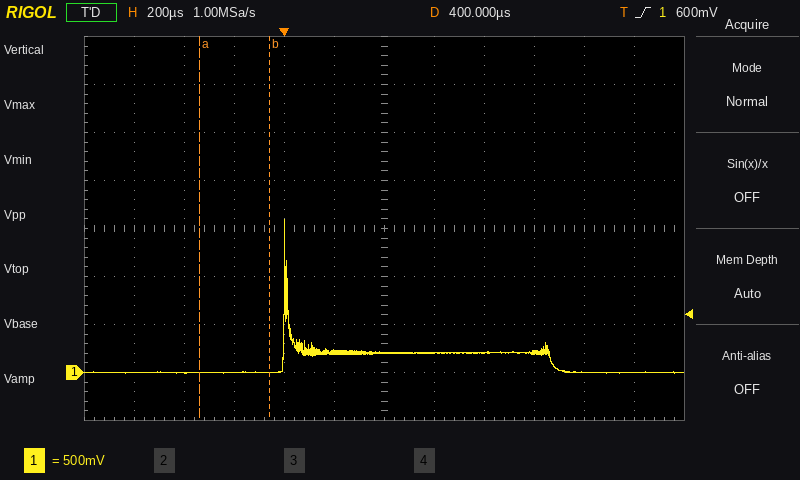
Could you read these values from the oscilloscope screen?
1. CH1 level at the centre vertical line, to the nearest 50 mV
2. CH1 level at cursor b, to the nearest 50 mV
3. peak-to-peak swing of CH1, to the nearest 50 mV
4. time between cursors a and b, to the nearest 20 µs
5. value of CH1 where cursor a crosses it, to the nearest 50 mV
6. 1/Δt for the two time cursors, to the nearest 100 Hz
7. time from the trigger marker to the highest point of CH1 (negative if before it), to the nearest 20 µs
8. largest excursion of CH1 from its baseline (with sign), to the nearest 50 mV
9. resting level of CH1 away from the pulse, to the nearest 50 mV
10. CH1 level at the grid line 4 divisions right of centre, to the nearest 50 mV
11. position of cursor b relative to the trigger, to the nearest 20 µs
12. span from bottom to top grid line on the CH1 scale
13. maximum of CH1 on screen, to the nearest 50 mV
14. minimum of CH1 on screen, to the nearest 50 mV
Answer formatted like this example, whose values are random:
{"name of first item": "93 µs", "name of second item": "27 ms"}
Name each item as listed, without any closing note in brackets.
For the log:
{"CH1 level at the centre vertical line, to the nearest 50 mV": "200 mV", "CH1 level at cursor b, to the nearest 50 mV": "0 mV", "peak-to-peak swing of CH1, to the nearest 50 mV": "1.60 V", "time between cursors a and b, to the nearest 20 µs": "280 µs", "value of CH1 where cursor a crosses it, to the nearest 50 mV": "0 mV", "1/Δt for the two time cursors, to the nearest 100 Hz": "3.6 kHz", "time from the trigger marker to the highest point of CH1 (negative if before it), to the nearest 20 µs": "0 µs", "largest excursion of CH1 from its baseline (with sign), to the nearest 50 mV": "+1.60 V", "resting level of CH1 away from the pulse, to the nearest 50 mV": "0 mV", "CH1 level at the grid line 4 divisions right of centre, to the nearest 50 mV": "0 mV", "position of cursor b relative to the trigger, to the nearest 20 µs": "-60 µs", "span from bottom to top grid line on the CH1 scale": "4 V", "maximum of CH1 on screen, to the nearest 50 mV": "1.60 V", "minimum of CH1 on screen, to the nearest 50 mV": "0 mV"}
